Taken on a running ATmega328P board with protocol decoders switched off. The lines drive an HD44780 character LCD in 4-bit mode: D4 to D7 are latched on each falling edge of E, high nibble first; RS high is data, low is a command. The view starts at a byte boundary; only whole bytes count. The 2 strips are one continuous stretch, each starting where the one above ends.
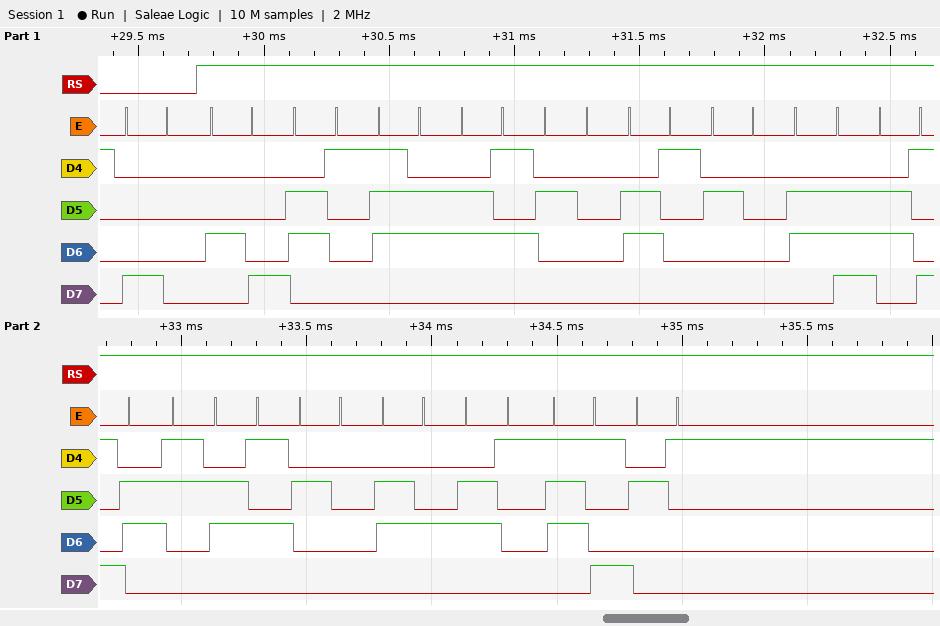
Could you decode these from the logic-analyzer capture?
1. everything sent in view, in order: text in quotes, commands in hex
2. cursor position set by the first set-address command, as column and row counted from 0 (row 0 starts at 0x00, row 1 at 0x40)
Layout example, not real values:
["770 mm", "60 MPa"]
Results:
["0x80 \"Have a nice day!\"", "column 0, row 0"]
